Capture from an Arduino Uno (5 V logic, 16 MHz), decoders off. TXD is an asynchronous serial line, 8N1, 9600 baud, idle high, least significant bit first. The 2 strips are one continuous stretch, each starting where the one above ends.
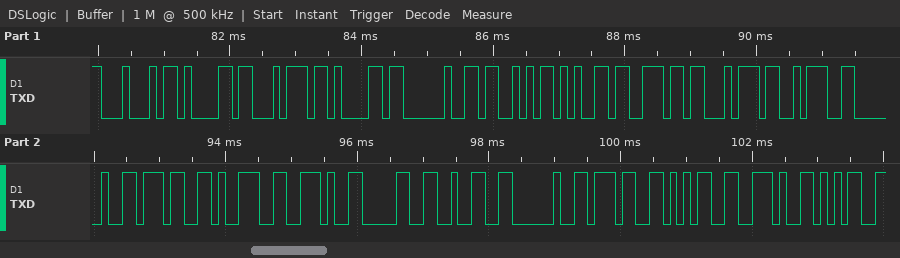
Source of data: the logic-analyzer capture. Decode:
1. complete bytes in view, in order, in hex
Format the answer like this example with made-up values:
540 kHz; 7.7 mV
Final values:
0x44 0x61 0x74 0x61 0x20 0x53 0x65 0x6E 0x74 0x3A 0x20 0x37 0x39 0x2E 0x30 0x32 0x20 0x37 0x35 0x2E 0x35
